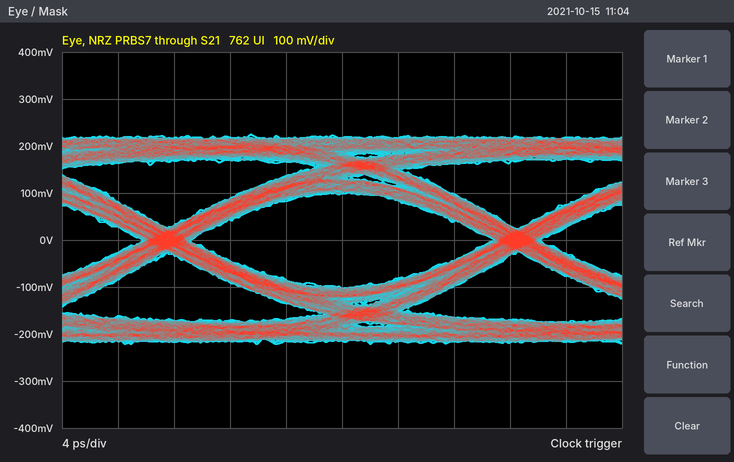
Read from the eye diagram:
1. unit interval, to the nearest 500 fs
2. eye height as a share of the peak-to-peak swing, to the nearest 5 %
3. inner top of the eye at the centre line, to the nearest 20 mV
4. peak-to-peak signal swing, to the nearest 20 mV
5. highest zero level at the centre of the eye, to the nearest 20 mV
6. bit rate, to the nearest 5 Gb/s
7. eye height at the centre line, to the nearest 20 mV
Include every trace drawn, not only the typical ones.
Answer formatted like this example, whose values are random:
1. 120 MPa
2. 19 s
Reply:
1. 25.0 ps
2. 45 %
3. 100 mV
4. 440 mV
5. -100 mV
6. 40 Gb/s
7. 200 mV
